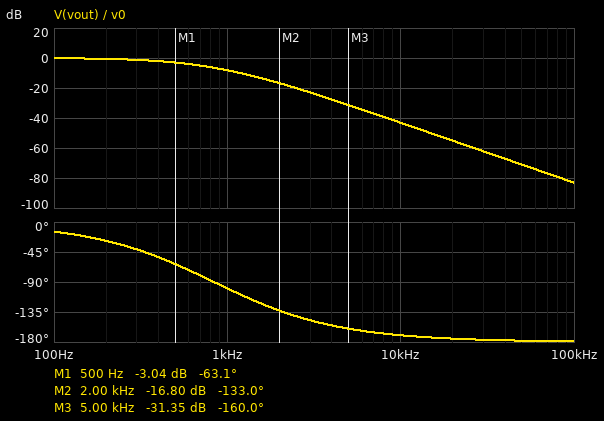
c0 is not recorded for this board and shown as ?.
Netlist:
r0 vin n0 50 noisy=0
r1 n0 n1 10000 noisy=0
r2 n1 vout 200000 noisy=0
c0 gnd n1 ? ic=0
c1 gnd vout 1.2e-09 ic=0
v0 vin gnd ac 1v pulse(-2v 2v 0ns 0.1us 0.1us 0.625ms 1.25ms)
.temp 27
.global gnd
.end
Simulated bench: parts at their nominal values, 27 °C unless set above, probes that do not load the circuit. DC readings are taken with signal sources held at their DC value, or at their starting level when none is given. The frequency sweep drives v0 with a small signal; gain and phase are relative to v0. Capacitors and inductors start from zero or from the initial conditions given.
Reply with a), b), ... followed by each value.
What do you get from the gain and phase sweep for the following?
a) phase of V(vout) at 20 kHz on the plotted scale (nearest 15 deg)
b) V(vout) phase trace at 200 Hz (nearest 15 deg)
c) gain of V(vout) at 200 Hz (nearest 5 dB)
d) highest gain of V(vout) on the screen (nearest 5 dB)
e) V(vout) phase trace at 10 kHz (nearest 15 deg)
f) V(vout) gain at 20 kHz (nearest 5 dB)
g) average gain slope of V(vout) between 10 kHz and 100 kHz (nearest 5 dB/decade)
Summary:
a) -180 deg
b) -30 deg
c) 0 dB
d) 0 dB
e) -165 deg
f) -55 dB
g) -40 dB/decade
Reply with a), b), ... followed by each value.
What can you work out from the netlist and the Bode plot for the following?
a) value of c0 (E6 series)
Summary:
a) 15 nF
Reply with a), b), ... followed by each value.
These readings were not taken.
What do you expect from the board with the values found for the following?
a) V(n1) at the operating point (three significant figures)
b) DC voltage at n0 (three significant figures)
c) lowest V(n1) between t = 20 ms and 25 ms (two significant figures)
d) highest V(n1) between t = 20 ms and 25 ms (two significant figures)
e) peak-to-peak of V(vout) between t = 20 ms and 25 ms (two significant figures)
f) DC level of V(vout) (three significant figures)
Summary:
a) -2.00 V
b) -2.00 V
c) -1.9 V
d) 1.9 V
e) 2.7 V
f) -2.00 V
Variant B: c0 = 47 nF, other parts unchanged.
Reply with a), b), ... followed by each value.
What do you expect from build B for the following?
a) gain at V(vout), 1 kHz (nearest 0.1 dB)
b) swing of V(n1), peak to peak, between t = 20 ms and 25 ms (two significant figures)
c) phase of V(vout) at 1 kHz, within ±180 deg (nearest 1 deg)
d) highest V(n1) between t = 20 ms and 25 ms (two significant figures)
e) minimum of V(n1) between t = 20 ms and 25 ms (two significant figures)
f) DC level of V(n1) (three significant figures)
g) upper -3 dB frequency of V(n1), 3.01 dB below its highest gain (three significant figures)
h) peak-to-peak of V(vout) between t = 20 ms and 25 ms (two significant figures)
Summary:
a) -15.2 dB
b) 2.3 V
c) -127 deg
d) 1.1 V
e) -1.1 V
f) -2.00 V
g) 327 Hz
h) 1.3 V
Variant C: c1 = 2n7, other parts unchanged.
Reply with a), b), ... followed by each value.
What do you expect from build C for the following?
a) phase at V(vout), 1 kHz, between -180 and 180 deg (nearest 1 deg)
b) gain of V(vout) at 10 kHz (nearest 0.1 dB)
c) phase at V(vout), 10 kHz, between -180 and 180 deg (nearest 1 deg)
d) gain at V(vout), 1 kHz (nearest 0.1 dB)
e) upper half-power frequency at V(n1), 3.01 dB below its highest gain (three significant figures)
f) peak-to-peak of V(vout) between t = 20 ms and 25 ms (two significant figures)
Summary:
a) -116 deg
b) -50.2 dB
c) -172 deg
d) -14.0 dB
e) 990 Hz
f) 1.5 V
